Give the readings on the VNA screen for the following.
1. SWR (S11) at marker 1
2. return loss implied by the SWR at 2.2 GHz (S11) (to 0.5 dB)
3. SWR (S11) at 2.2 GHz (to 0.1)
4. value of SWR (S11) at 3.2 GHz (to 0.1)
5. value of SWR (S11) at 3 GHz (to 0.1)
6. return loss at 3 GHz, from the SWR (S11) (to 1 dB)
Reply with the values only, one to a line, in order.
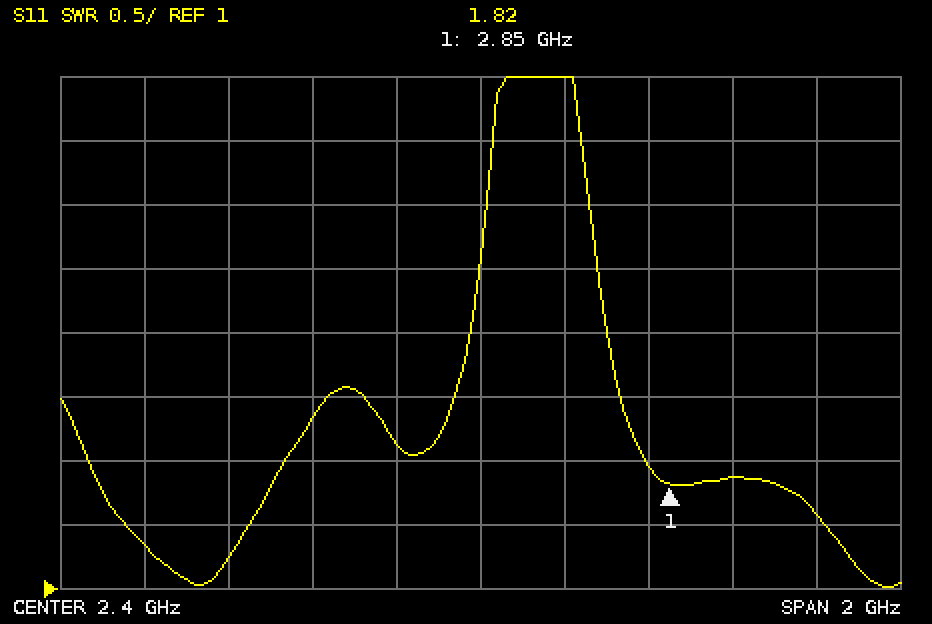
1.82
9.0 dB
2.1
1.6
1.9
10 dB
